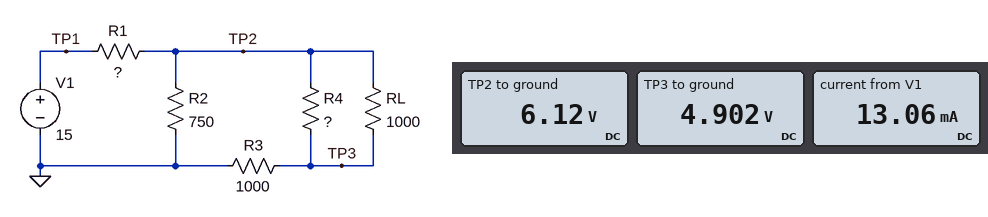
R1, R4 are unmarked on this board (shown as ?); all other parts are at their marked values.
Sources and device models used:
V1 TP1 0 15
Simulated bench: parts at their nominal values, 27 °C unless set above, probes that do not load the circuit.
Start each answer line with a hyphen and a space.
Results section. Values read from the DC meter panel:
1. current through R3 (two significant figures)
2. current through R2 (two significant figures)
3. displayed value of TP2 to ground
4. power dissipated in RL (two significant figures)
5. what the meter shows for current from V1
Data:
- 4.9 mA
- 8.2 mA
- 6.12 V
- 1.5 mW
- 13.06 mA
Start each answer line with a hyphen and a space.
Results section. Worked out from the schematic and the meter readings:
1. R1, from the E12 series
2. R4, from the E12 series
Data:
- 680 Ω
- 330 Ω
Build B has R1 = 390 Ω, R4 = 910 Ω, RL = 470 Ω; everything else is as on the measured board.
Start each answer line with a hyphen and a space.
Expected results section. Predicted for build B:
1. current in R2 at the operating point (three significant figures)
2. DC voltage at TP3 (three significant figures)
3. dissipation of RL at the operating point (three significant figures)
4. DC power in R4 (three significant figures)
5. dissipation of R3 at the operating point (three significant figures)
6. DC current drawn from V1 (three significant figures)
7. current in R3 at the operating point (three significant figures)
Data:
- 11.0 mA
- 6.30 V
- 8.11 mW
- 4.19 mW
- 39.7 mW
- 17.3 mA
- 6.30 mA
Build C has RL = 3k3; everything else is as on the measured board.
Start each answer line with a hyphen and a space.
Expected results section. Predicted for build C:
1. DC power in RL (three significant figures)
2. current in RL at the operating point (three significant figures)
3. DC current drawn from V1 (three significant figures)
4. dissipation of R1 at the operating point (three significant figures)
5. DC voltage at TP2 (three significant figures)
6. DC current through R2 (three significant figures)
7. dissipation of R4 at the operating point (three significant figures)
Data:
- 615 µW
- 432 µA
- 13.0 mA
- 115 mW
- 6.17 V
- 8.23 mA
- 6.15 mW
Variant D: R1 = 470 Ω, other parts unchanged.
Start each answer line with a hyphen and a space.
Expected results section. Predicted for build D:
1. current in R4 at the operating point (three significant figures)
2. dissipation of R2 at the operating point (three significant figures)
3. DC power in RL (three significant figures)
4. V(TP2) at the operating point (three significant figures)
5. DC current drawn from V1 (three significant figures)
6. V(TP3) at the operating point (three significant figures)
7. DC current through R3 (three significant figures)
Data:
- 4.51 mA
- 74.8 mW
- 2.22 mW
- 7.49 V
- 16.0 mA
- 6.00 V
- 6.00 mA
